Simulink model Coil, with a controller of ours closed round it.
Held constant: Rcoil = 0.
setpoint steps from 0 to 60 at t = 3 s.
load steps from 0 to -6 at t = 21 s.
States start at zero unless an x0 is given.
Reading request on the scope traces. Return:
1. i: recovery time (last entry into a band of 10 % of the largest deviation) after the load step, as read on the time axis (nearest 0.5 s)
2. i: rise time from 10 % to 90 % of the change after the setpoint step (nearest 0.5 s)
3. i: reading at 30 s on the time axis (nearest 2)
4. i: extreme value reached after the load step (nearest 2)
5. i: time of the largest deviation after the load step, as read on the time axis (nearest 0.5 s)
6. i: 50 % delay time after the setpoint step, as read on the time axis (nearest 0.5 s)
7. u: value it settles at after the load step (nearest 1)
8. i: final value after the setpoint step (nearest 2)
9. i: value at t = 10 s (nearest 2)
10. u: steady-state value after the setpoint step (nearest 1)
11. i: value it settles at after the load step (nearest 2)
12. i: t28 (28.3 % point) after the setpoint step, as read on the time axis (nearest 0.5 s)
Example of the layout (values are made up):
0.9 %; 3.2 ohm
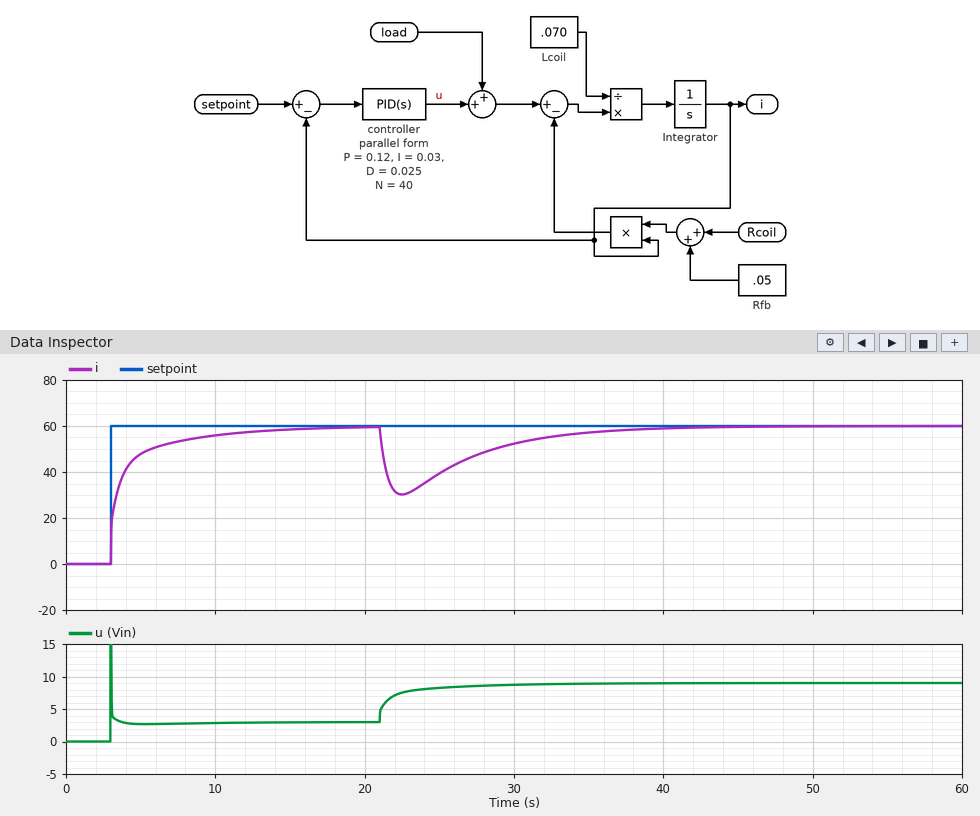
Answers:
35.0 s; 5.0 s; 52; 30; 22.5 s; 3.5 s; 9; 60; 56; 3; 60; 3.0 s
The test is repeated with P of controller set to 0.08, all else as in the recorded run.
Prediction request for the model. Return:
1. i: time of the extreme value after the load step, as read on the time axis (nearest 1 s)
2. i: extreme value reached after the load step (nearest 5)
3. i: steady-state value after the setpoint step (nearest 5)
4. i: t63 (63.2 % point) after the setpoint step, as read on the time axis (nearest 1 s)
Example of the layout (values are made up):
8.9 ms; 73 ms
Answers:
23 s; 25; 60; 4 s
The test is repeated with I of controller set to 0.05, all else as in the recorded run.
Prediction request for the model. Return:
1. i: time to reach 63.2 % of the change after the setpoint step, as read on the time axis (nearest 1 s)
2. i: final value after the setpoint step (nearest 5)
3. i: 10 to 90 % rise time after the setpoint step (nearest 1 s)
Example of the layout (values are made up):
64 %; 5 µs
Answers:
4 s; 60; 3 s
